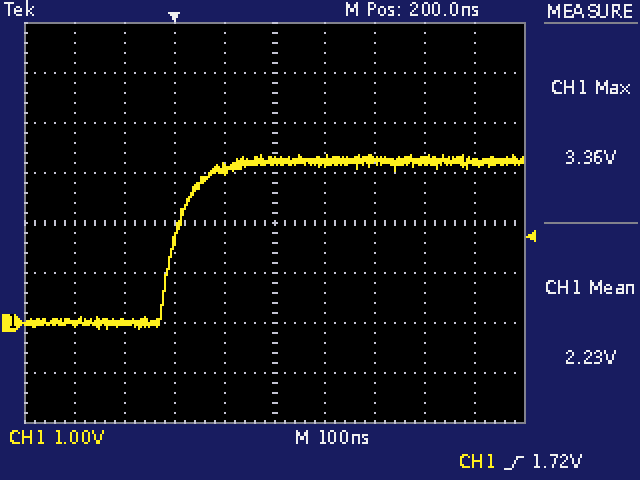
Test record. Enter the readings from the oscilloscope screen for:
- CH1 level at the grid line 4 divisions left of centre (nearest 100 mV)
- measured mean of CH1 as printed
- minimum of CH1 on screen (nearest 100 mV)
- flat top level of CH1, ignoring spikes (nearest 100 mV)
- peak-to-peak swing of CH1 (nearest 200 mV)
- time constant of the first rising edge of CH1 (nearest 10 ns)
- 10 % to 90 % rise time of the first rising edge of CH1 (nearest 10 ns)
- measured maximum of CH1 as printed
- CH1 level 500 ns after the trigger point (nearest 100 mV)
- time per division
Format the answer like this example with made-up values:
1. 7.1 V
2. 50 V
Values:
1. 0.0 V
2. 2.23 V
3. -100 mV
4. 3.2 V
5. 3.4 V
6. 40 ns
7. 90 ns
8. 3.36 V
9. 3.2 V
10. 100 ns
